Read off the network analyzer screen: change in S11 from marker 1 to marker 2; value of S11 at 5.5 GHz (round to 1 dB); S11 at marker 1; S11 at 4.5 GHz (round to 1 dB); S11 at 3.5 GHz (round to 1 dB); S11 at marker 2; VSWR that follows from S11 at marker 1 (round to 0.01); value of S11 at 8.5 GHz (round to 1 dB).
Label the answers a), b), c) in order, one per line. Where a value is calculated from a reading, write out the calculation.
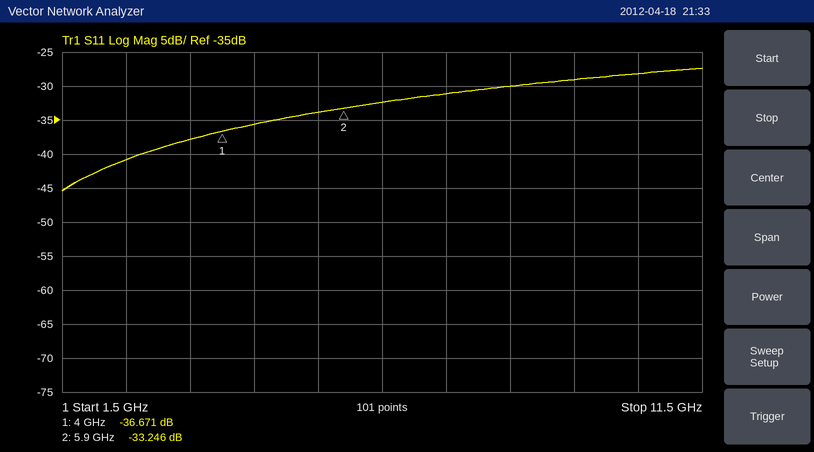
a) -33.246 − (-36.671) = 3.425 dB
b) -34 dB
c) -36.671 dB
d) -36 dB
e) -38 dB
f) -33.246 dB
g) (1 + 0.0147)/(1 − 0.0147) ≈ 1.03
h) -30 dB
